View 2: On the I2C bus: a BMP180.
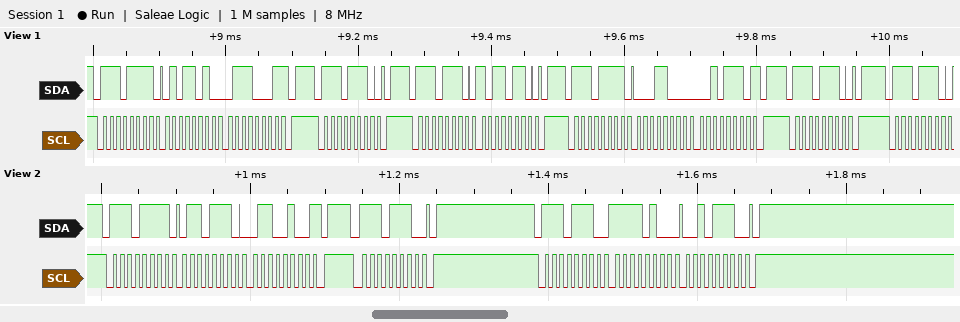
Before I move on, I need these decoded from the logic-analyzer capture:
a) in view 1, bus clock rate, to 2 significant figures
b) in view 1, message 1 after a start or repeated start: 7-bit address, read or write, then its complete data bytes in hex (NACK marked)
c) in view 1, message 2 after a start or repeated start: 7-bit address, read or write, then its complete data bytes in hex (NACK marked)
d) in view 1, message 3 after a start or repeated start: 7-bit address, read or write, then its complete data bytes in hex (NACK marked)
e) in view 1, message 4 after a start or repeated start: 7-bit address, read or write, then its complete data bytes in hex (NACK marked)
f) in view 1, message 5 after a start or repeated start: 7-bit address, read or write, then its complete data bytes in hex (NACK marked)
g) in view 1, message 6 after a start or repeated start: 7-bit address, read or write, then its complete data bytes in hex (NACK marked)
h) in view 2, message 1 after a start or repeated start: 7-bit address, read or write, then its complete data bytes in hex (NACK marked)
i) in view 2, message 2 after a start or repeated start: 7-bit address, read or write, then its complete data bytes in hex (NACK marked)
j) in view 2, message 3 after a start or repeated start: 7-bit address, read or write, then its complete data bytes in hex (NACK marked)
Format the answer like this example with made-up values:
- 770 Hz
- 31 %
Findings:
- 100 kHz
- 0x77 read: 5A 71 NACK
- 0x77 write
- 0x77 write: B6
- 0x77 read: 18 2E NACK
- 0x77 write
- 0x77 write
- 0x77 read: 6E 64 NACK
- 0x77 write
- 0x77 write: F4 2E
